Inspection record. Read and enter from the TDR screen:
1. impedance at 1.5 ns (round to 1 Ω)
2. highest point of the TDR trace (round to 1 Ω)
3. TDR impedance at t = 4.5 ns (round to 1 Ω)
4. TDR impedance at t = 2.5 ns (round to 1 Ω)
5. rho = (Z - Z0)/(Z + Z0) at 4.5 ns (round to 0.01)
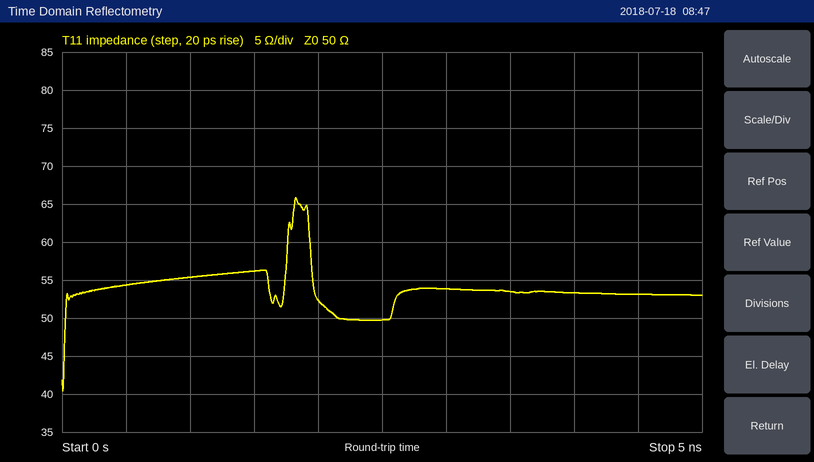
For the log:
56 Ω
66 Ω
53 Ω
50 Ω
+0.03
